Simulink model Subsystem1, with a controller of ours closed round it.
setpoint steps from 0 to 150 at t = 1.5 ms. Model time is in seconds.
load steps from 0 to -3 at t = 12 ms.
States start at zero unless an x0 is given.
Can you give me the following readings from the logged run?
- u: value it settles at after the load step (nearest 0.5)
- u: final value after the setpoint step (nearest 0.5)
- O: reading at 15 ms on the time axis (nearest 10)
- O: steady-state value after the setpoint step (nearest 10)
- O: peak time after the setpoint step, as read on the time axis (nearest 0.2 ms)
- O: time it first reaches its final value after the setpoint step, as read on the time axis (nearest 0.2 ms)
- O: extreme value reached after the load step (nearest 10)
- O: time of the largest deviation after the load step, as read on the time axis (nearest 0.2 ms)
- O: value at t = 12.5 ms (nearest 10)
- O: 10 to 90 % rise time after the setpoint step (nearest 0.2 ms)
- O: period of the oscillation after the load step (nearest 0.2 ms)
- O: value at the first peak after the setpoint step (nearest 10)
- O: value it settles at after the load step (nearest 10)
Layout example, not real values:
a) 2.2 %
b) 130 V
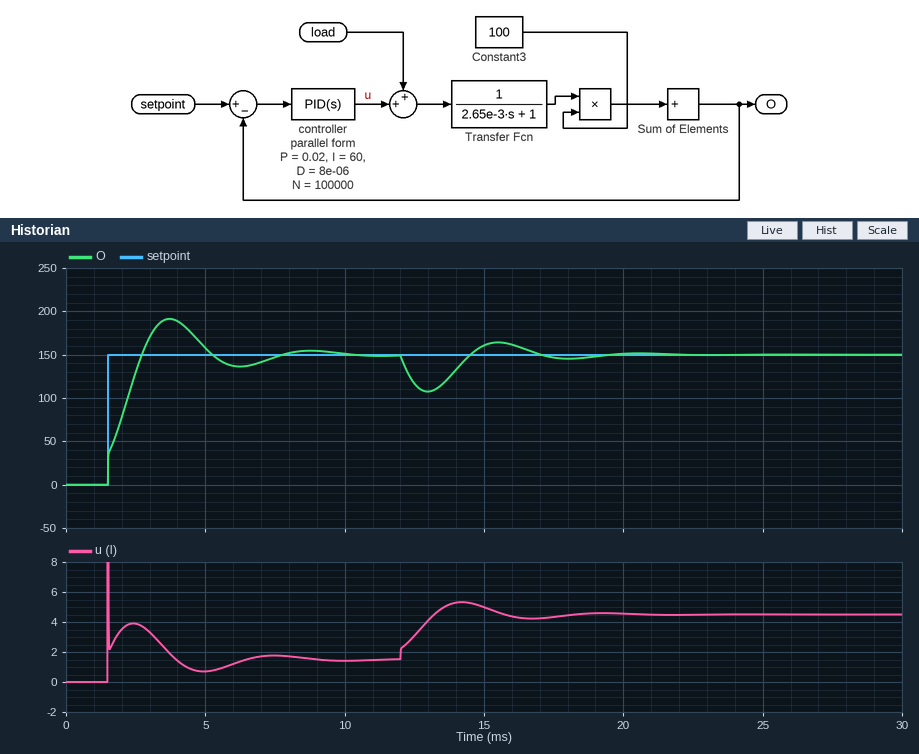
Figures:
a) 4.5
b) 1.5
c) 160
d) 150
e) 3.8 ms
f) 2.8 ms
g) 110
h) 13.0 ms
i) 120
j) 1.0 ms
k) 5.0 ms
l) 190
m) 150
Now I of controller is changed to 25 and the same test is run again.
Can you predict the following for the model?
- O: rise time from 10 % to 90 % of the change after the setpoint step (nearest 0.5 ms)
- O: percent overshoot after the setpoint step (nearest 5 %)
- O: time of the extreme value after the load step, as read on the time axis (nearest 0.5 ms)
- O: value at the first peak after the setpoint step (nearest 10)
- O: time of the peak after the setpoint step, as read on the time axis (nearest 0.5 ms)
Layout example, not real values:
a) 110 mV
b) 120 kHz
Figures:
a) 1.5 ms
b) 15 %
c) 13.5 ms
d) 170
e) 5.0 ms
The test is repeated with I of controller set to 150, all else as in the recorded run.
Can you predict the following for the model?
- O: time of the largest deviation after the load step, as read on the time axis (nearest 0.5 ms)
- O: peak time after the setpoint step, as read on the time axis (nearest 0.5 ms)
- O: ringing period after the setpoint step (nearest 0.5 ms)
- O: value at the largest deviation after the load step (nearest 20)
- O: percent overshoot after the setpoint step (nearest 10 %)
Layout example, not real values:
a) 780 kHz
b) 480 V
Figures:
a) 12.5 ms
b) 3.0 ms
c) 3.0 ms
d) 120
e) 40 %
